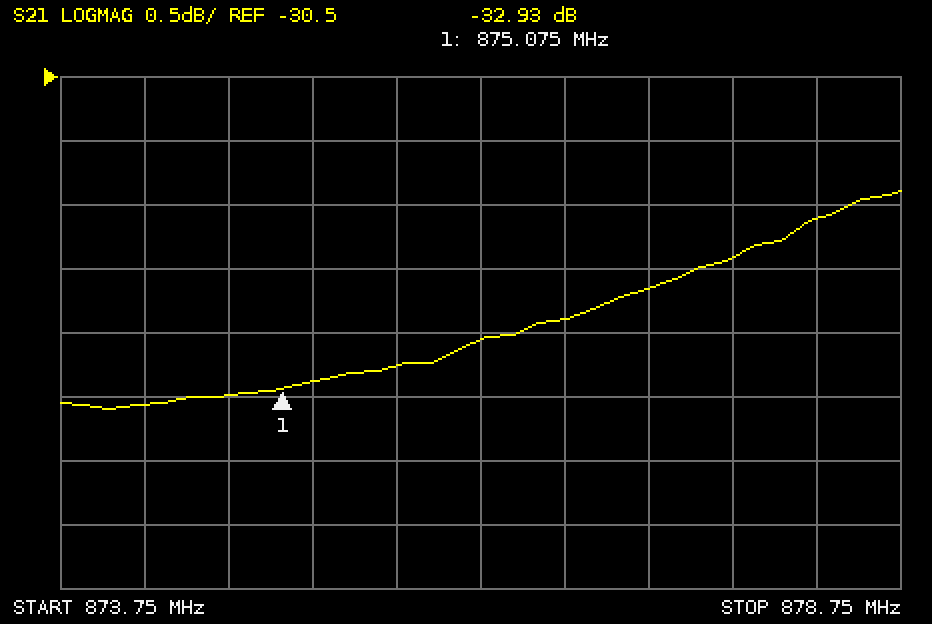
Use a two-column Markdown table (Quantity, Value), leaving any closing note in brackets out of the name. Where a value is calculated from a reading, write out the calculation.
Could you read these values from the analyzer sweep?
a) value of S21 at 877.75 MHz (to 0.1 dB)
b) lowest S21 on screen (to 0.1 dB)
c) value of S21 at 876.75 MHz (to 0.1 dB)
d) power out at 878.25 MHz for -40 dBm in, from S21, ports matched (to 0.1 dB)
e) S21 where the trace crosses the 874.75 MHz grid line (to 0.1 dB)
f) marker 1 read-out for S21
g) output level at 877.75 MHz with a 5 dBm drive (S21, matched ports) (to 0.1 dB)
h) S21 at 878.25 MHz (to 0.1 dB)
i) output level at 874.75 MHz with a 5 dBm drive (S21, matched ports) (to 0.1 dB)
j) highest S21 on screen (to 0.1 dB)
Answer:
| Quantity | Value |
|---|---|
| value of S21 at 877.75 MHz | -31.9 dB |
| lowest S21 on screen | -33.1 dB |
| value of S21 at 876.75 MHz | -32.4 dB |
| power out at 878.25 MHz for -40 dBm in, from S21, ports matched | -40 dBm + (-31.6 dB) = -71.6 dBm |
| S21 where the trace crosses the 874.75 MHz grid line | -33.0 dB |
| marker 1 read-out for S21 | -32.93 dB |
| output level at 877.75 MHz with a 5 dBm drive (S21, matched ports) | 5 dBm + (-31.9 dB) = -26.9 dBm |
| S21 at 878.25 MHz | -31.6 dB |
| output level at 874.75 MHz with a 5 dBm drive (S21, matched ports) | 5 dBm + (-33.0 dB) = -28.0 dBm |
| highest S21 on screen | -31.4 dB |
